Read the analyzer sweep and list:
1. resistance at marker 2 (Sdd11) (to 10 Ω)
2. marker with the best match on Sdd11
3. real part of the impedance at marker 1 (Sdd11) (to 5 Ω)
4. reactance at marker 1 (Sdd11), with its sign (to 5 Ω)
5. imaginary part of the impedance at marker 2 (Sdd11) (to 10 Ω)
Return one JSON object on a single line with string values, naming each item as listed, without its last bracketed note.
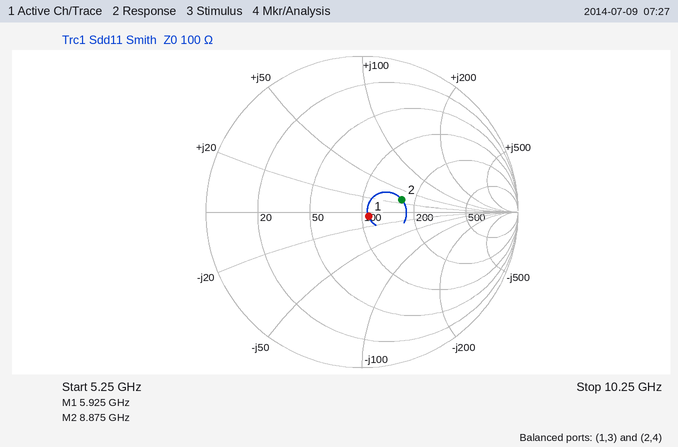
{"resistance at marker 2 (Sdd11)": "170 Ω", "marker with the best match on Sdd11": "marker 1", "real part of the impedance at marker 1 (Sdd11)": "110 Ω", "reactance at marker 1 (Sdd11), with its sign": "-5 Ω", "imaginary part of the impedance at marker 2 (Sdd11)": "+30 Ω"}
